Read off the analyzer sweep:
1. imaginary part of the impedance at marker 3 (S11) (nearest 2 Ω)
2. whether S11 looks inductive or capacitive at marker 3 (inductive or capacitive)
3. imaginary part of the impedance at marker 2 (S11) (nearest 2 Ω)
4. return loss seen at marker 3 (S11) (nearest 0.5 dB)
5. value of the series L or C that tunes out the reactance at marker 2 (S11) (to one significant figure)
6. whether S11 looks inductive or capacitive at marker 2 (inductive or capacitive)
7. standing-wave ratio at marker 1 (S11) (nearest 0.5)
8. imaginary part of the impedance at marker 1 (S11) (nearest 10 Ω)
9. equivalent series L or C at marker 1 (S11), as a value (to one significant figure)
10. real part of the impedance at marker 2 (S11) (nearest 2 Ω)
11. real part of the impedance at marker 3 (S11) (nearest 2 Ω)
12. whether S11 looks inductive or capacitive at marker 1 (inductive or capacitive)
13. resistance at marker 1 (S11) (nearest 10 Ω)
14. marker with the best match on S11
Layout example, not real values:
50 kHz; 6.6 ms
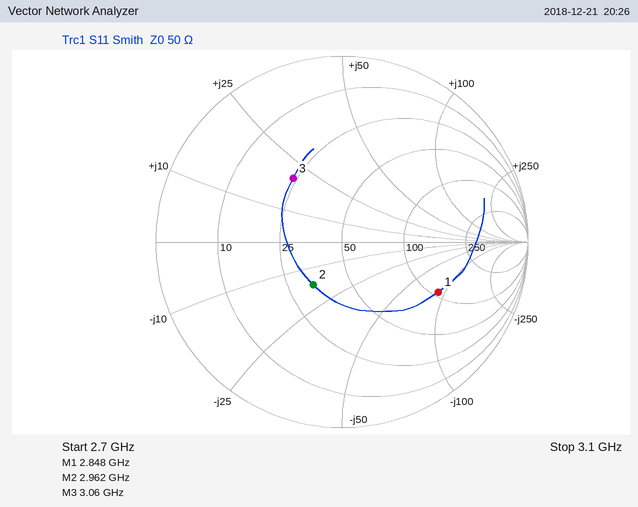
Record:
+20 Ω; inductive; -16 Ω; 7.5 dB; 900 pH; capacitive; 4.0; -90 Ω; 600 fF; 34 Ω; 24 Ω; capacitive; 110 Ω; marker 2
